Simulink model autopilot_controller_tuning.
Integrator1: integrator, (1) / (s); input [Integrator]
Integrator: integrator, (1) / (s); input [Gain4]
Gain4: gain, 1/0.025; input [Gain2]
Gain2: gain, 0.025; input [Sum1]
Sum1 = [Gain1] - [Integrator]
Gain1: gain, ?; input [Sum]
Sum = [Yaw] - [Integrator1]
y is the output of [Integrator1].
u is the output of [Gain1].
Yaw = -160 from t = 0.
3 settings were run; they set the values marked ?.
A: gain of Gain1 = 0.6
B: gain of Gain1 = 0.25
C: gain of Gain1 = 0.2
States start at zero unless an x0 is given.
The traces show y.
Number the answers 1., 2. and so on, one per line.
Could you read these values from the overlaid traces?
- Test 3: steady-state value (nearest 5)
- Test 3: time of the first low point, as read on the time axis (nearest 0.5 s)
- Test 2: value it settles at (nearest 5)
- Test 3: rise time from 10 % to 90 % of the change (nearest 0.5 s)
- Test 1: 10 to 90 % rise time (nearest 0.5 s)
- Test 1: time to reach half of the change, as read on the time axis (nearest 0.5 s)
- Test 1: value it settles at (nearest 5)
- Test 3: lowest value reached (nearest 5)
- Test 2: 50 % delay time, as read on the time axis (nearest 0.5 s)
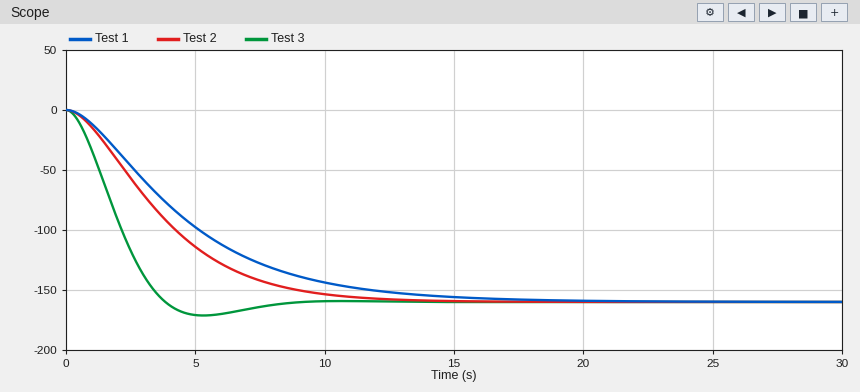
1. -160
2. 5.5 s
3. -160
4. 2.5 s
5. 9.0 s
6. 4.0 s
7. -160
8. -170
9. 3.5 s
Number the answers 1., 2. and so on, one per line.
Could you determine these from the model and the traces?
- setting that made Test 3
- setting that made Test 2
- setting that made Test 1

1. A
2. B
3. C
